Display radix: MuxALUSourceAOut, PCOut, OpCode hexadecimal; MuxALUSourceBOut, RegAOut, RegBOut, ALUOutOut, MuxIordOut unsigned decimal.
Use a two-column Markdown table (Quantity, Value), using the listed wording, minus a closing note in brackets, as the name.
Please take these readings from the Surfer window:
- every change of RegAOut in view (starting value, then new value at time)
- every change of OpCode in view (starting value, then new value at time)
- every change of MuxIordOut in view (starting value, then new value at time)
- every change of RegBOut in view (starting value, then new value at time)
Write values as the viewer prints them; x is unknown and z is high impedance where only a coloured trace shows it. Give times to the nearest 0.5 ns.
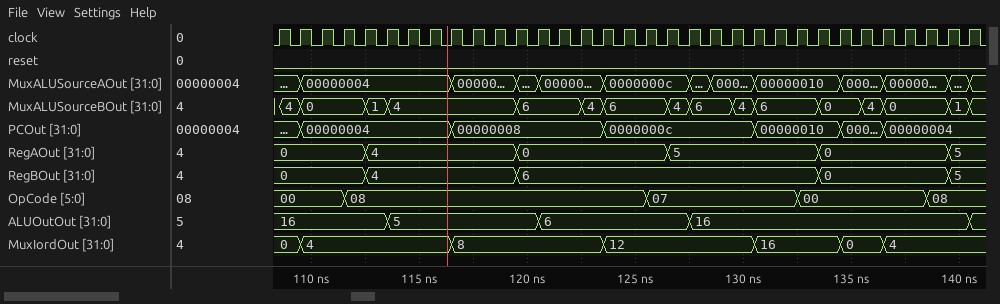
| Quantity | Value |
|---|---|
| every change of RegAOut in view | 0, 4 at 112.5 ns, 0 at 119.5 ns, 5 at 126.5 ns, 0 at 133.5 ns, 5 at 139.5 ns |
| every change of OpCode in view | 00, 08 at 111.5 ns, 07 at 125.5 ns, 00 at 132.5 ns, 08 at 138.5 ns |
| every change of MuxIordOut in view | 0, 4 at 109.5 ns, 8 at 116.5 ns, 12 at 123.5 ns, 16 at 130.5 ns, 0 at 134.5 ns, 4 at 136.5 ns |
| every change of RegBOut in view | 0, 4 at 112.5 ns, 6 at 119.5 ns, 0 at 133.5 ns, 5 at 139.5 ns |
